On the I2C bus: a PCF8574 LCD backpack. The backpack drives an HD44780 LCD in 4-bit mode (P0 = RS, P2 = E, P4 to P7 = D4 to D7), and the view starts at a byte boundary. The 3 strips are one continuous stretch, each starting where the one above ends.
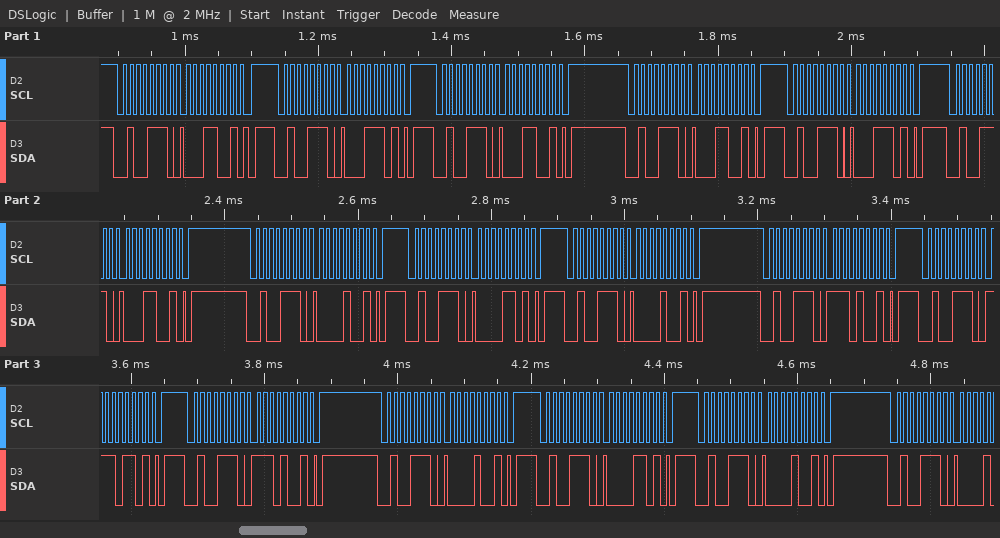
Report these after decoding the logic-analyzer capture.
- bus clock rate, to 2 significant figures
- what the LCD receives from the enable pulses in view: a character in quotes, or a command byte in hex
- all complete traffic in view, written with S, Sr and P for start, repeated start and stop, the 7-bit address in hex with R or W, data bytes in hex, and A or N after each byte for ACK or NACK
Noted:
100 kHz
data 0x11 data 0x0E
S 27W A 19 A P S 27W A 1D A P S 27W A 19 A P S 27W A 19 A P S 27W A 1D A P S 27W A 19 A P S 27W A 09 A P S 27W A 0D A P S 27W A 09 A P S 27W A E9 A P S 27W A ED A P S 27W A E9 A P S 27W A 09 A P S 27W A 0D A P S 27W A 09 A P S 27W A
